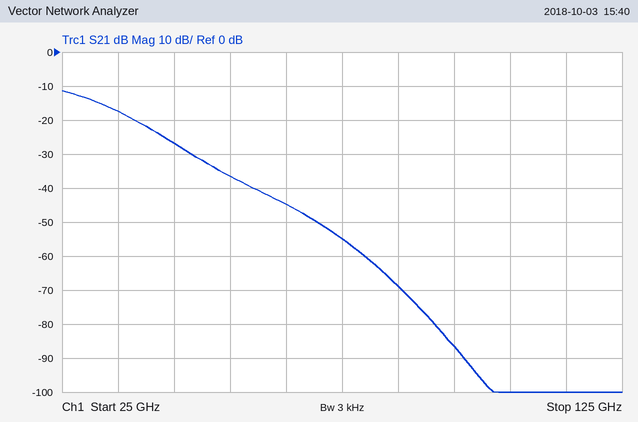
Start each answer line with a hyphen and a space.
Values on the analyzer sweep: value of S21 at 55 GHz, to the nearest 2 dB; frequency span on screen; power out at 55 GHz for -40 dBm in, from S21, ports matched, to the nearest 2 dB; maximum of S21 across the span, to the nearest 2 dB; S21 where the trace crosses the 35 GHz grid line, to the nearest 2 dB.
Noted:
- -36 dB
- 100 GHz
- -76 dBm
- -12 dB
- -18 dB
